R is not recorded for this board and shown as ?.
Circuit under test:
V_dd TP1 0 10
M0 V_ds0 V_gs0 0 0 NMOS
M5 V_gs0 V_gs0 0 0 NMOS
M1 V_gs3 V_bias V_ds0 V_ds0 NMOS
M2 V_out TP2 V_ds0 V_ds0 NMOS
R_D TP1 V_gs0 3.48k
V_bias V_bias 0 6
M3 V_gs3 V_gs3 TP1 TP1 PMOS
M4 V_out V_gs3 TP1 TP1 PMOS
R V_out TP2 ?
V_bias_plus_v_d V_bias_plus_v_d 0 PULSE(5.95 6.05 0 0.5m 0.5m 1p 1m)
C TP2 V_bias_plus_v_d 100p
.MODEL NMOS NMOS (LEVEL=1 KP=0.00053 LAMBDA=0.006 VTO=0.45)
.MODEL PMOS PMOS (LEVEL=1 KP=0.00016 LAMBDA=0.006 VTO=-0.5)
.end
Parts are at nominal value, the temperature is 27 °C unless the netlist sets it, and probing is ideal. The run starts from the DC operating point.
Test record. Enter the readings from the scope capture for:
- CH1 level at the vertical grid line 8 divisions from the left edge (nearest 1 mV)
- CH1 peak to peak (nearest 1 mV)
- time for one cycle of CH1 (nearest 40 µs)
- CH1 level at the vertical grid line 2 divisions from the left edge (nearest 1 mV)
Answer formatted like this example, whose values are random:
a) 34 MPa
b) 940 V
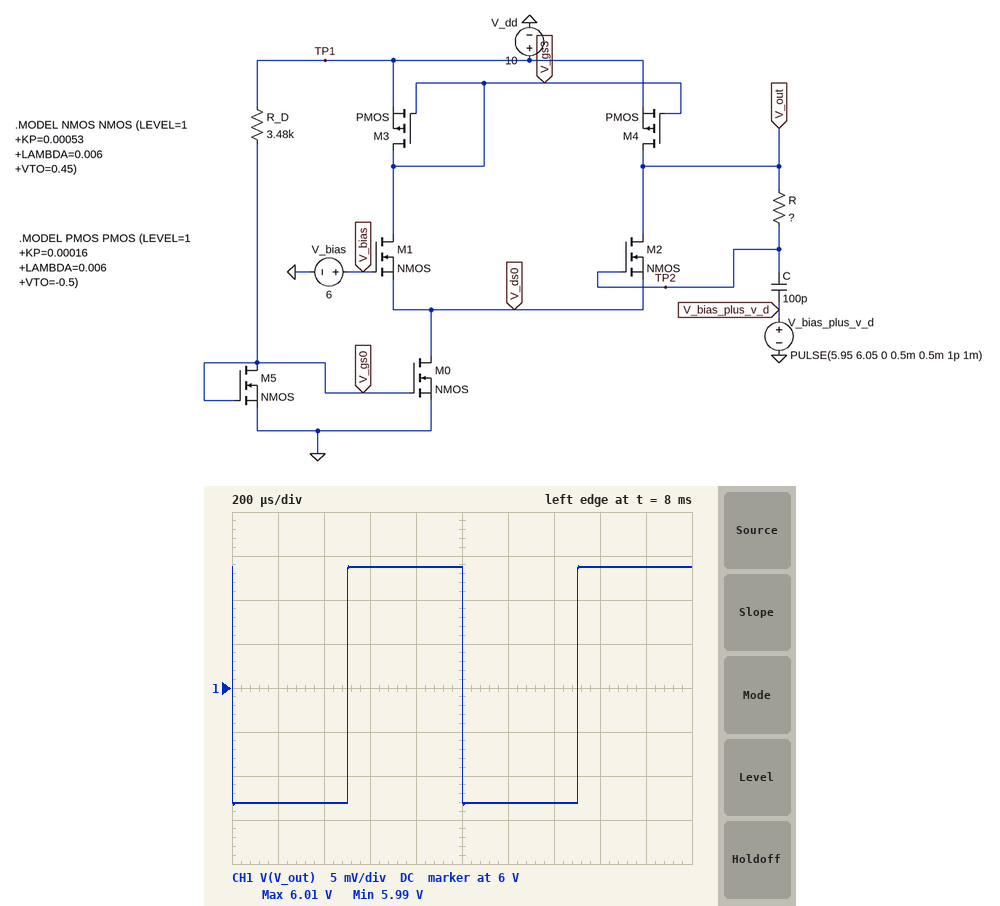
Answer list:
a) 6.014 V
b) 27 mV
c) 1.00 ms
d) 5.987 V
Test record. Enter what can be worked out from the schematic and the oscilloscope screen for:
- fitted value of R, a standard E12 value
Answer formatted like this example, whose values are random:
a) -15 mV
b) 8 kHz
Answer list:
a) 680 kΩ
